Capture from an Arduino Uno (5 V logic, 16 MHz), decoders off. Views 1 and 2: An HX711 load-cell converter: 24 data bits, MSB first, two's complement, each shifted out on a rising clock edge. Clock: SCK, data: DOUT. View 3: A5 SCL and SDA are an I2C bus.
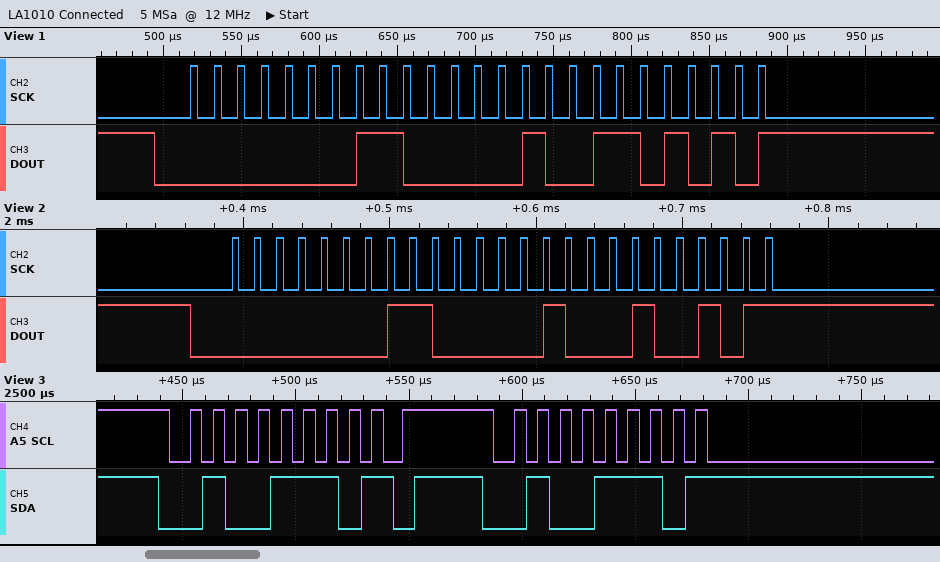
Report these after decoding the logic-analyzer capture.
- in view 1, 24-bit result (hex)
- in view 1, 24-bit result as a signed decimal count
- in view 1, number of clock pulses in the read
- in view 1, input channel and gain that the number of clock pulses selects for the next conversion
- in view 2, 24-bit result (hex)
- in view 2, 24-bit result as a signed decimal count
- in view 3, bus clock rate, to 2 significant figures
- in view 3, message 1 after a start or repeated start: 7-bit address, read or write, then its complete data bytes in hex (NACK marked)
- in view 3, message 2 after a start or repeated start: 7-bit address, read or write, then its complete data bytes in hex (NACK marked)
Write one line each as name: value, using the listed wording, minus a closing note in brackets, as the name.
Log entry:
in view 1, 24-bit result: 0x01826A
in view 1, 24-bit result as a signed decimal count: 98922
in view 1, number of clock pulses in the read: 25
in view 1, input channel and gain that the number of clock pulses selects for the next conversion: channel A, gain 128
in view 2, 24-bit result: 0x018225
in view 2, 24-bit result as a signed decimal count: 98853
in view 3, bus clock rate, to 2 significant figures: 100 kHz
in view 3, message 1 after a start or repeated start: 7-bit address, read or write, then its complete data bytes in hex: 0x27 write NACK
in view 3, message 2 after a start or repeated start: 7-bit address, read or write, then its complete data bytes in hex: 0x27 write NACK
